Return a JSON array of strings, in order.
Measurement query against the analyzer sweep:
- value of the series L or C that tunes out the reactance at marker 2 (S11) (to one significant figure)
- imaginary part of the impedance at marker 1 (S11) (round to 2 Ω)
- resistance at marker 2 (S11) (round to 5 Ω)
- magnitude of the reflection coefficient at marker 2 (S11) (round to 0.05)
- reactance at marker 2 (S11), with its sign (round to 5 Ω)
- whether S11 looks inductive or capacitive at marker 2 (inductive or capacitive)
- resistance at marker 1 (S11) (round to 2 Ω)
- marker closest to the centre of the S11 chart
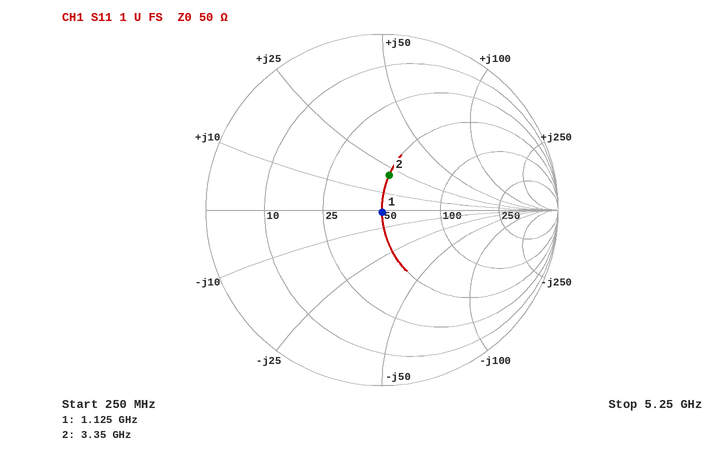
["2 pF", "-2 Ω", "50 Ω", "0.20", "+20 Ω", "inductive", "50 Ω", "marker 1"]
